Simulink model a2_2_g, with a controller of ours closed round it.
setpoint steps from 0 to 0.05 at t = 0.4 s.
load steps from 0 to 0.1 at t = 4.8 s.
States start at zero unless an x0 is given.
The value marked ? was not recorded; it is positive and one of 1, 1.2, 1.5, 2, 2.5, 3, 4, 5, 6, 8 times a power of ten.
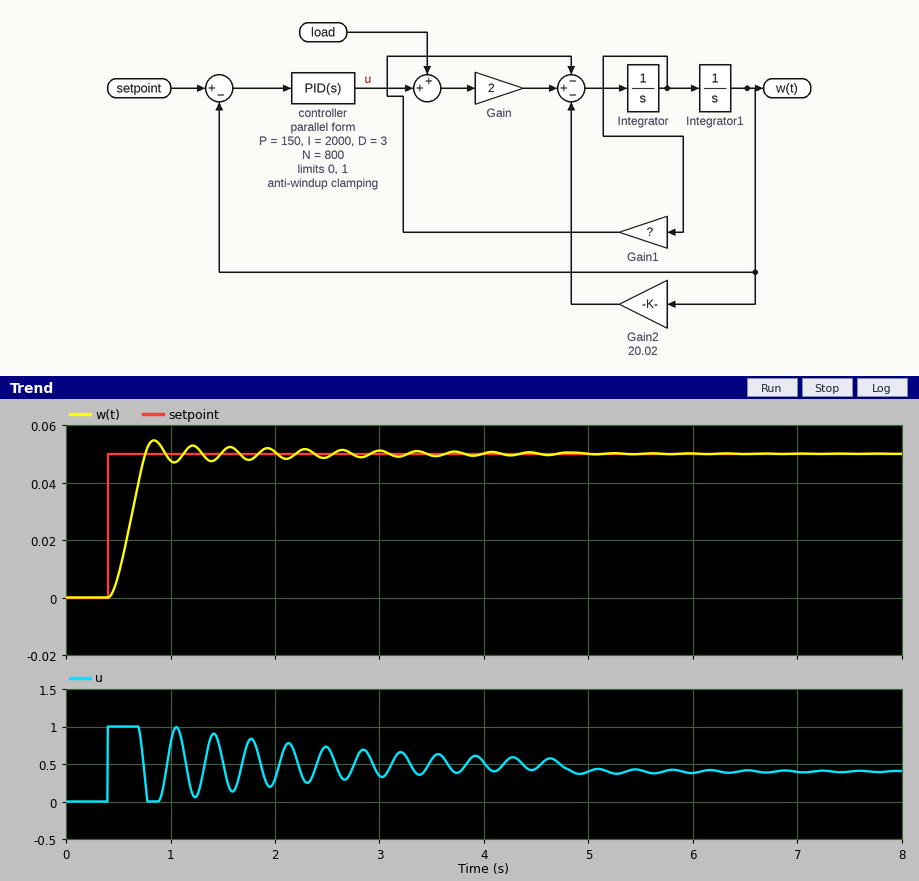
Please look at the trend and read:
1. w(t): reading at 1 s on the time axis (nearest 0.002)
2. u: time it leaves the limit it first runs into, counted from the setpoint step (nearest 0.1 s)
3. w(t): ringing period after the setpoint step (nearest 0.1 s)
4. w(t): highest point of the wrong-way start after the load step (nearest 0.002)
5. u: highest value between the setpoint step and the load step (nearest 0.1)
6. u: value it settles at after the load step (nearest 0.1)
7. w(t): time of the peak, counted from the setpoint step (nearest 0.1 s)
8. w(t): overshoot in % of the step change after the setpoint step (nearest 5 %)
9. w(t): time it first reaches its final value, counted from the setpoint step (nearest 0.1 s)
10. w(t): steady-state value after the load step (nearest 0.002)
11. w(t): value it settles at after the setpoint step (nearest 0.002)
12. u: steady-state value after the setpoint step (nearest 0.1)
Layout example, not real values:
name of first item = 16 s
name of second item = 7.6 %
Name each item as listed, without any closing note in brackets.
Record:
w(t): reading at 1 s on the time axis = 0.048
u: time it leaves the limit it first runs into, counted from the setpoint step = 0.3 s
w(t): ringing period after the setpoint step = 0.4 s
w(t): highest point of the wrong-way start after the load step = 0.050
u: highest value between the setpoint step and the load step = 1.0
u: value it settles at after the load step = 0.4
w(t): time of the peak, counted from the setpoint step = 0.4 s
w(t): overshoot in % of the step change after the setpoint step = 10 %
w(t): time it first reaches its final value, counted from the setpoint step = 0.4 s
w(t): steady-state value after the load step = 0.050
w(t): value it settles at after the setpoint step = 0.050
u: steady-state value after the setpoint step = 0.5
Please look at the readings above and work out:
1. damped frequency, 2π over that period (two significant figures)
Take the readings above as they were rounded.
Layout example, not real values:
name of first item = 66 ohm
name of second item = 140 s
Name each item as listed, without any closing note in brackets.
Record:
damped frequency, 2π over that period = 16 rad/s
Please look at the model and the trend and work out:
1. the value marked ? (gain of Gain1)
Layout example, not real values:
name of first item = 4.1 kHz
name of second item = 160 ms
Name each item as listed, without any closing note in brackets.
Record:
the value marked ? = 8
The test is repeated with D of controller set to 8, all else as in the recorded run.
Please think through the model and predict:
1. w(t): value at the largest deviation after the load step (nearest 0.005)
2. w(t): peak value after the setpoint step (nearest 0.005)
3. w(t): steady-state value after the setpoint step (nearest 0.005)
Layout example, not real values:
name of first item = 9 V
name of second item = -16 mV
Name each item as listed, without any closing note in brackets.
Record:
w(t): value at the largest deviation after the load step = 0.050
w(t): peak value after the setpoint step = 0.055
w(t): steady-state value after the setpoint step = 0.050
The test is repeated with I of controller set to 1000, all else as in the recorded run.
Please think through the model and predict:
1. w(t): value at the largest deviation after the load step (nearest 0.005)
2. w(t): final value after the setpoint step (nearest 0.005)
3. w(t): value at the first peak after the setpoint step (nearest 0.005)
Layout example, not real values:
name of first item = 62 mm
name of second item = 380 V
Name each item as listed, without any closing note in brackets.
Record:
w(t): value at the largest deviation after the load step = 0.050
w(t): final value after the setpoint step = 0.050
w(t): value at the first peak after the setpoint step = 0.055
